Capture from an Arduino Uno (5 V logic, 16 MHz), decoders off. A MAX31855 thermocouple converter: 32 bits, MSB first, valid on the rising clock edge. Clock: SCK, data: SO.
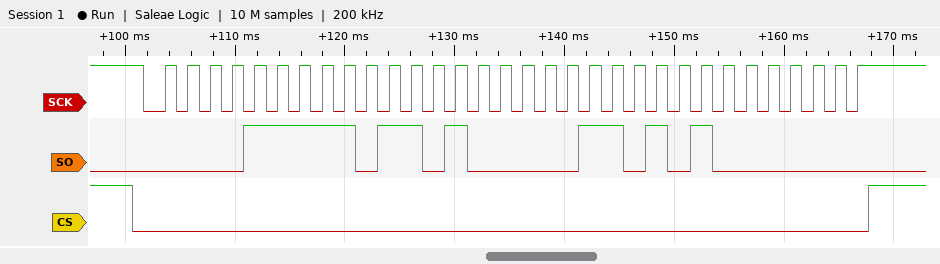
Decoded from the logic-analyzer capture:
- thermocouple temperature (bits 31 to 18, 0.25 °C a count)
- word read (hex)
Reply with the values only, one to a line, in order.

251.25 °C
0x0FB41A80
